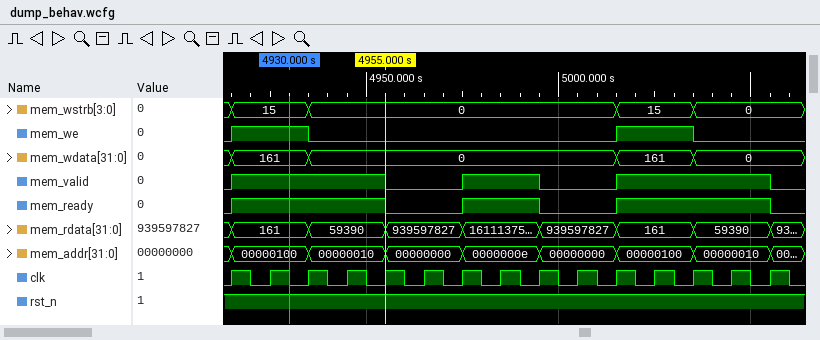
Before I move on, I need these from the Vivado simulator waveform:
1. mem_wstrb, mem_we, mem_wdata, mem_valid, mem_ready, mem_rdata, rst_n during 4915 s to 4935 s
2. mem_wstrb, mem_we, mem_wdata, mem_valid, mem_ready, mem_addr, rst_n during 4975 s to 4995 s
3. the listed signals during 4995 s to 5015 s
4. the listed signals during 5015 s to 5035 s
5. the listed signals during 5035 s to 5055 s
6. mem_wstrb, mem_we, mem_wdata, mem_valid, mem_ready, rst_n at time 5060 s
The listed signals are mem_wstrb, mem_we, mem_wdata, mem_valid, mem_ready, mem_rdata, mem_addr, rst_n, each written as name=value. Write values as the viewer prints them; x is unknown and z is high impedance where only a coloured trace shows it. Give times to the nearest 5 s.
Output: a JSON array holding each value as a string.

["mem_wstrb=15, mem_we=1, mem_wdata=161, mem_valid=1, mem_ready=1, mem_rdata=161, rst_n=1", "mem_wstrb=0, mem_we=0, mem_wdata=0, mem_valid=1, mem_ready=1, mem_addr=0000000e, rst_n=1", "mem_wstrb=0, mem_we=0, mem_wdata=0, mem_valid=0, mem_ready=0, mem_rdata=939597827, mem_addr=00000000, rst_n=1", "mem_wstrb=15, mem_we=1, mem_wdata=161, mem_valid=1, mem_ready=1, mem_rdata=161, mem_addr=00000100, rst_n=1", "mem_wstrb=0, mem_we=0, mem_wdata=0, mem_valid=1, mem_ready=1, mem_rdata=59390, mem_addr=00000010, rst_n=1", "mem_wstrb=0, mem_we=0, mem_wdata=0, mem_valid=0, mem_ready=0, rst_n=1"]
